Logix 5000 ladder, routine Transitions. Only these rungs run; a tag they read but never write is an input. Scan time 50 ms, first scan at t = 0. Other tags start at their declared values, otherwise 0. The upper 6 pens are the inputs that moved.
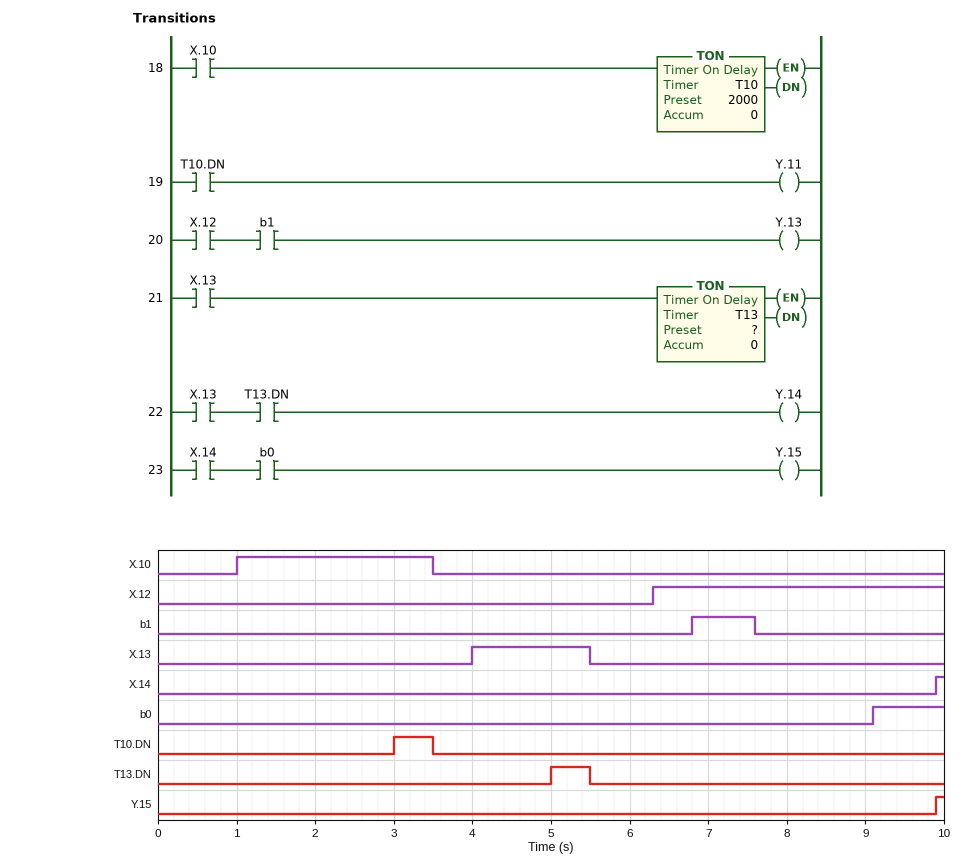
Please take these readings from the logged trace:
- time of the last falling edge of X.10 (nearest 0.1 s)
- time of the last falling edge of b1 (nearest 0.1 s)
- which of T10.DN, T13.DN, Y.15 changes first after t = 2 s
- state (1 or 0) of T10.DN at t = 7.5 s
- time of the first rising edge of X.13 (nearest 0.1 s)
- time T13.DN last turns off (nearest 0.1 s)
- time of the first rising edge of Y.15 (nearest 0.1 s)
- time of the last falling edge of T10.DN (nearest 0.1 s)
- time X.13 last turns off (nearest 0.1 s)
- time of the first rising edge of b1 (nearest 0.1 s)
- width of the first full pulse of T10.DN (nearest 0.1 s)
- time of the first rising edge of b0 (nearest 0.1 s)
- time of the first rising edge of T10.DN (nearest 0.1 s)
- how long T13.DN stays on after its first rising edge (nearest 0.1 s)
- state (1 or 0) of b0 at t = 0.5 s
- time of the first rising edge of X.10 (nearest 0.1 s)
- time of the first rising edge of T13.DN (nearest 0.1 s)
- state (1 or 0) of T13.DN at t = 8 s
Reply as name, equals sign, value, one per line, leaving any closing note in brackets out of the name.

time of the last falling edge of X.10 = 3.5 s
time of the last falling edge of b1 = 7.6 s
which of T10.DN, T13.DN, Y.15 changes first after t = 2 s = T10.DN
state (1 or 0) of T10.DN at t = 7.5 s = 0
time of the first rising edge of X.13 = 4.0 s
time T13.DN last turns off = 5.5 s
time of the first rising edge of Y.15 = 9.9 s
time of the last falling edge of T10.DN = 3.5 s
time X.13 last turns off = 5.5 s
time of the first rising edge of b1 = 6.8 s
width of the first full pulse of T10.DN = 0.5 s
time of the first rising edge of b0 = 9.1 s
time of the first rising edge of T10.DN = 3.0 s
how long T13.DN stays on after its first rising edge = 0.5 s
state (1 or 0) of b0 at t = 0.5 s = 0
time of the first rising edge of X.10 = 1.0 s
time of the first rising edge of T13.DN = 5.0 s
state (1 or 0) of T13.DN at t = 8 s = 0
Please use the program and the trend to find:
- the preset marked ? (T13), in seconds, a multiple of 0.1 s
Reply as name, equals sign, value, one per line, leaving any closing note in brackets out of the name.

the preset marked ? (T13), in seconds, a multiple of 0.1 s = 1.0 s
